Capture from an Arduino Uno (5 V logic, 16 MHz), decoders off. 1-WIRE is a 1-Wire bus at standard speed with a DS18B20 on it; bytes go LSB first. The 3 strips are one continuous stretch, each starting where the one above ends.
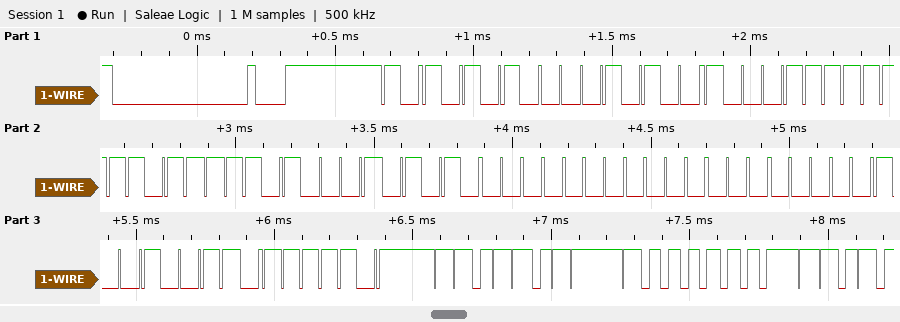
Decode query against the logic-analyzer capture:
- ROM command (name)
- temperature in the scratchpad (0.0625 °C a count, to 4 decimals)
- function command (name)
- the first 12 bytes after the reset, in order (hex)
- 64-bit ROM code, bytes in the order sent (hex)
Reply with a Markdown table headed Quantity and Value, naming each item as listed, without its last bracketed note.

| Quantity | Value |
|---|---|
| ROM command | Match ROM |
| temperature in the scratchpad | 29.6875 °C |
| function command | Read Scratchpad |
| the first 12 bytes after the reset, in order | 55 28 F1 EF 8B 0A 00 00 C9 BE DB 01 |
| 64-bit ROM code, bytes in the order sent | 28 F1 EF 8B 0A 00 00 C9 |
